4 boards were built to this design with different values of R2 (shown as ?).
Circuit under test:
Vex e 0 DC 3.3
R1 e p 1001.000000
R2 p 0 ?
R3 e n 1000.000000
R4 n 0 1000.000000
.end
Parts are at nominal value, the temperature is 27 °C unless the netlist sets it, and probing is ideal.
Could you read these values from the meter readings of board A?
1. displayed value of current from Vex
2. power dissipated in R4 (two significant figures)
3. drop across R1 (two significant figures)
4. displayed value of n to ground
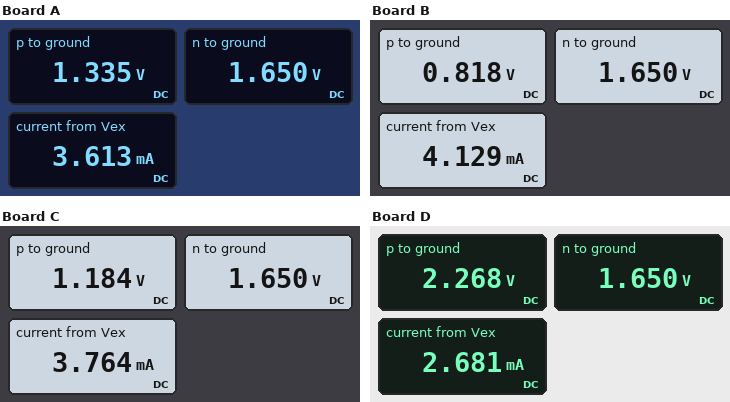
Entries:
3.613 mA
2.7 mW
2.0 V
1.650 V
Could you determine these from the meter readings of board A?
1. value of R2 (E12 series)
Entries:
680 Ω
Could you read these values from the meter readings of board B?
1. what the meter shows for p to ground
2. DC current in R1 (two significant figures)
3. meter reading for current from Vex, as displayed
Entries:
0.818 V
2.5 mA
4.129 mA
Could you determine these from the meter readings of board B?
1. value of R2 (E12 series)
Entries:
330 Ω
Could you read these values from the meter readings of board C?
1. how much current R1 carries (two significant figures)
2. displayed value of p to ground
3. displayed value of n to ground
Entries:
2.1 mA
1.184 V
1.650 V
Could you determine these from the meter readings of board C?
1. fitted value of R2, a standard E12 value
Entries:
560 Ω
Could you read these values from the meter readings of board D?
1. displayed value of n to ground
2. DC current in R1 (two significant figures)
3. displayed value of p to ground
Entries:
1.650 V
1.0 mA
2.268 V
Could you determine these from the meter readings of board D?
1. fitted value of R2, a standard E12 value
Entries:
2.2 kΩ
